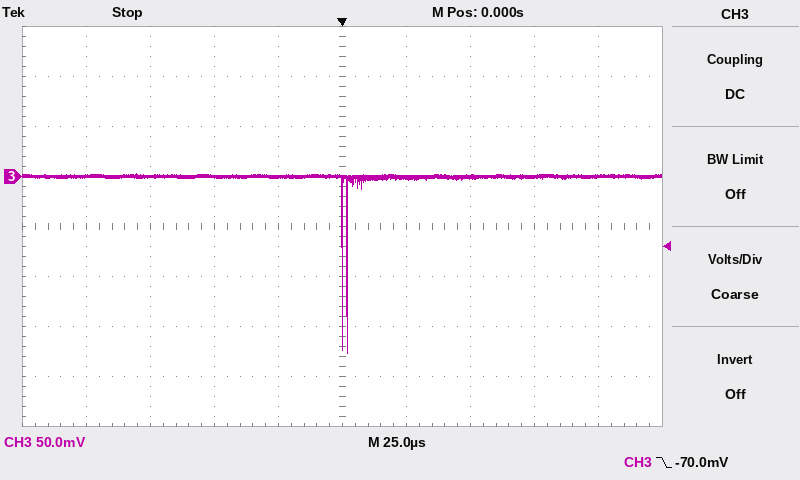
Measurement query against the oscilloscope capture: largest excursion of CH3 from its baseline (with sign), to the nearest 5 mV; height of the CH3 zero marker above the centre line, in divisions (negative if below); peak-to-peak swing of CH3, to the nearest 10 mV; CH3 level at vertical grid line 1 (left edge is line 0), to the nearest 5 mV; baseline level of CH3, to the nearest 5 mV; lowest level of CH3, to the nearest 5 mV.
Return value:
-175 mV
+1.0 div
180 mV
0 mV
0 mV
-175 mV
